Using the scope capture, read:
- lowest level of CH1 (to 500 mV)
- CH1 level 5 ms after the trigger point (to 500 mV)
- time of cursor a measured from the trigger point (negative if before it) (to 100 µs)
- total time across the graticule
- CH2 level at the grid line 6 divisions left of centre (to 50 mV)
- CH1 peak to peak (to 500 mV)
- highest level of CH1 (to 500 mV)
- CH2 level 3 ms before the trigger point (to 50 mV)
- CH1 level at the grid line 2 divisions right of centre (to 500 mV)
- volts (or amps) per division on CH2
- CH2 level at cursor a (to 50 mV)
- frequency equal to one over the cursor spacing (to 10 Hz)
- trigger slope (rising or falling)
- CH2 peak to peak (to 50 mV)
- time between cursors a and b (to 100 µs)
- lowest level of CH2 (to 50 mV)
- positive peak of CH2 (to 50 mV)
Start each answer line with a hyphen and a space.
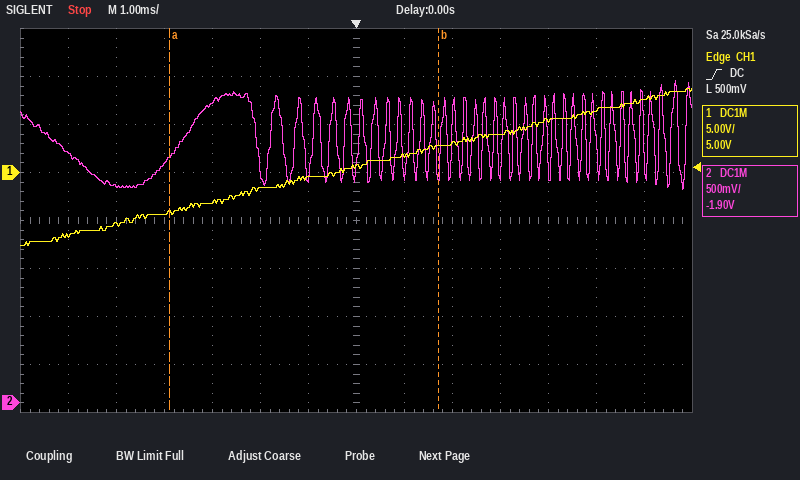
- -7.5 V
- 6.5 V
- -3.9 ms
- 14 ms
- 2.60 V
- 16.5 V
- 9.0 V
- 3.15 V
- 3.0 V
- 500 mV
- 2.55 V
- 180 Hz
- rising
- 1.15 V
- 5.6 ms
- 2.20 V
- 3.35 V
